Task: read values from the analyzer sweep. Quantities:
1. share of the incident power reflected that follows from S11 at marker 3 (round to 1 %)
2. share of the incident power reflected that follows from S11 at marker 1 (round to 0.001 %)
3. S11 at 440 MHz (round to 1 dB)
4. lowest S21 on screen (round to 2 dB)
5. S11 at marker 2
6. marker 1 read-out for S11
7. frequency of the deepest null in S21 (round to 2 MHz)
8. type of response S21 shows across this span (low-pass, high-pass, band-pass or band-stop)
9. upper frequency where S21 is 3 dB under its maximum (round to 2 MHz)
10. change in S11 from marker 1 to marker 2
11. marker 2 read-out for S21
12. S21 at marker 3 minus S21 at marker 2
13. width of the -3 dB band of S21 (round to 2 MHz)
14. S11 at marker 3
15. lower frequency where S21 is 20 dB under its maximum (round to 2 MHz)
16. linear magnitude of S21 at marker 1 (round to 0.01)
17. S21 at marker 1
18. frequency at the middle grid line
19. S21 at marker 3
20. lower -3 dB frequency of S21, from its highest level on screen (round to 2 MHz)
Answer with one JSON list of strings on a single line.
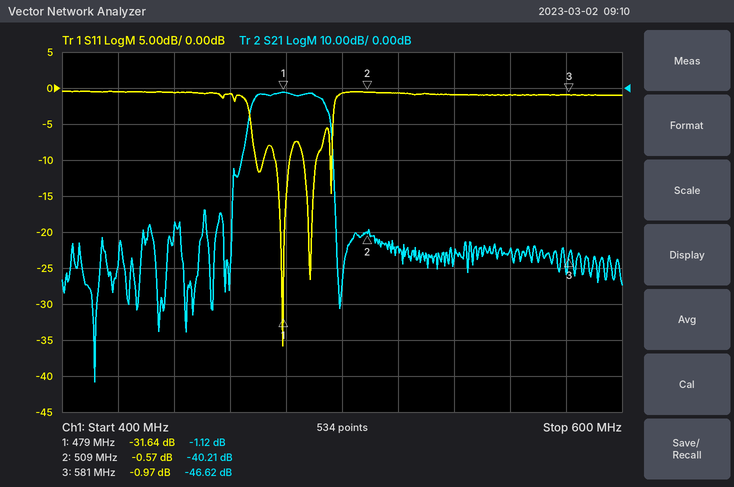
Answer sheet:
["80 %", "0.069 %", "-1 dB", "-82 dB", "-0.57 dB", "-31.64 dB", "412 MHz", "band-pass", "494 MHz", "31.07 dB", "-40.21 dB", "-6.41 dB", "26 MHz", "-0.97 dB", "464 MHz", "0.88", "-1.12 dB", "500 MHz", "-46.62 dB", "468 MHz"]
